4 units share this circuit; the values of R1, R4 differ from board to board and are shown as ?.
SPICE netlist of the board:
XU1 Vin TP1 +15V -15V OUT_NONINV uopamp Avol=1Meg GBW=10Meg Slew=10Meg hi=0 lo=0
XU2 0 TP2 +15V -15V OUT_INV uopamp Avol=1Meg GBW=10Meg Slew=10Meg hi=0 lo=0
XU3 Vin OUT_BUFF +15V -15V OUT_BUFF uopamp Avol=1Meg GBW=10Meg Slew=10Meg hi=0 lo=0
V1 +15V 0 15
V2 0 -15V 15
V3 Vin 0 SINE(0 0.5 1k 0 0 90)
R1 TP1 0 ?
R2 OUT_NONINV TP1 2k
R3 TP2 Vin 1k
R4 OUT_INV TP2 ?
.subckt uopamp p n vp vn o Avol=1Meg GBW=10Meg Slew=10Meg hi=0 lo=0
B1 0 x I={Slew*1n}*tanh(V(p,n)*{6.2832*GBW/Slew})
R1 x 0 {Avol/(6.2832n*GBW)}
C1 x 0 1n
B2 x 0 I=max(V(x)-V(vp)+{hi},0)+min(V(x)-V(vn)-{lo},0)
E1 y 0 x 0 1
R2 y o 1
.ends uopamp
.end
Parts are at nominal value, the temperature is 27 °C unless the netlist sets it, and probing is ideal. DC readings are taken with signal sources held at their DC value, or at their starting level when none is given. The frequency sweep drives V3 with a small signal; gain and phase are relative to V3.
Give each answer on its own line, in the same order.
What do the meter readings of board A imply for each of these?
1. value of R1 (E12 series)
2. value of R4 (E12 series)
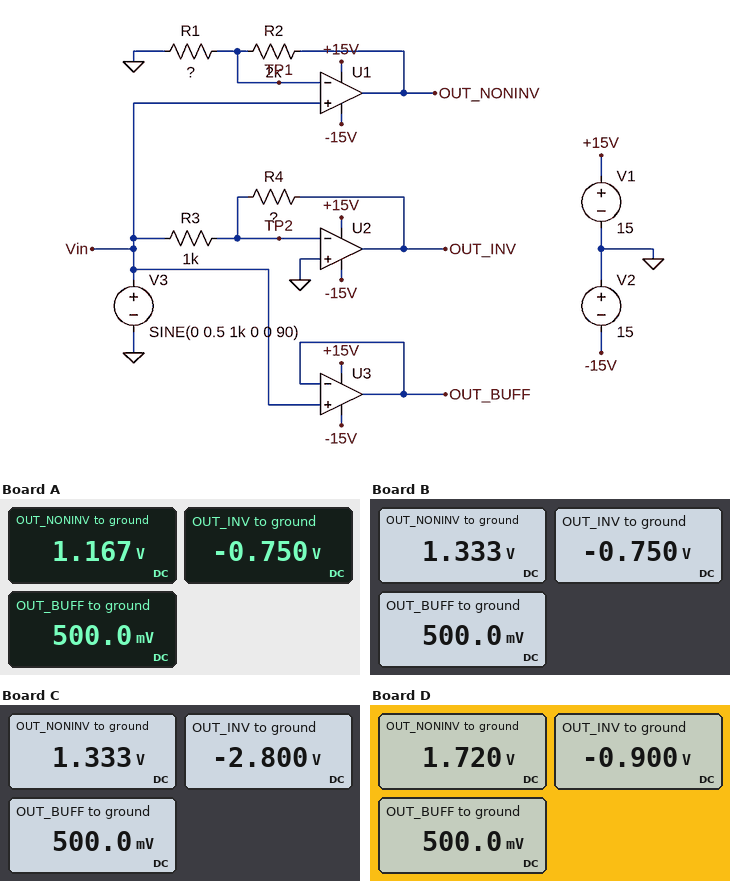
1.5 kΩ
1.5 kΩ
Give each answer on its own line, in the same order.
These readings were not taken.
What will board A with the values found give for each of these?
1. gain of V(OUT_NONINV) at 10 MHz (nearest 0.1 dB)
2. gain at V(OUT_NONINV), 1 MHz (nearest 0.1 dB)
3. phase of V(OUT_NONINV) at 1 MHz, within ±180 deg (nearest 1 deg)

-0.7 dB
7.1 dB
-13 deg
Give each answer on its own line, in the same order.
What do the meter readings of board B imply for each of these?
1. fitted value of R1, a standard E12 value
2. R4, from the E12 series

1.2 kΩ
1.5 kΩ
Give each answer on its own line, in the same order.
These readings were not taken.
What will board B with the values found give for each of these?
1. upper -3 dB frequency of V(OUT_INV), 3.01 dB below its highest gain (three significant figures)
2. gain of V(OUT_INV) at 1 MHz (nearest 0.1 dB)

4.00 MHz
3.3 dB
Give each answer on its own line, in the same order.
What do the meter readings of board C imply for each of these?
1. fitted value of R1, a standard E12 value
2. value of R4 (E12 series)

1.2 kΩ
5.6 kΩ
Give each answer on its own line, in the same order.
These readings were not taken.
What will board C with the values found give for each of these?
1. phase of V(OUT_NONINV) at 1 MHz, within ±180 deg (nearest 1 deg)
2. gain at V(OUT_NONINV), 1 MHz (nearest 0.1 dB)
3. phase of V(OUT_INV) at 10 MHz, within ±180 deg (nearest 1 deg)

-15 deg
8.2 dB
99 deg
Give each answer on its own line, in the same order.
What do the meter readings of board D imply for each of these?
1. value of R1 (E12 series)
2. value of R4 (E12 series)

820 Ω
1.8 kΩ
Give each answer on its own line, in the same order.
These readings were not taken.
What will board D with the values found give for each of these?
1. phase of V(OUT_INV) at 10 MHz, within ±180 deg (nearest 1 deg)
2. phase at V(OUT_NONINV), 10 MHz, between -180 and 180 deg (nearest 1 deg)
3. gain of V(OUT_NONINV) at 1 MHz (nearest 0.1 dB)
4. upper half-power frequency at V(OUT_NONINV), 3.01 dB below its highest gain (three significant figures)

110 deg
-74 deg
10.2 dB
2.91 MHz
